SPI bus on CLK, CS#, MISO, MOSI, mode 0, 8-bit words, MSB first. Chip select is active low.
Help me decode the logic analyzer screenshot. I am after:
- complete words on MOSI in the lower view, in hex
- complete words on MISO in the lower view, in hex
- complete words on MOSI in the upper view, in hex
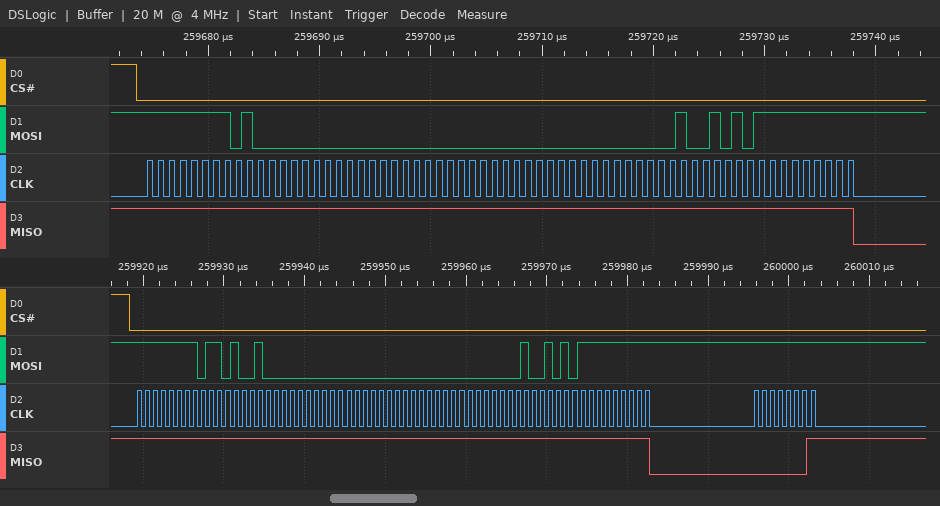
FF, 69, 00, 00, 00, 00, 95, FF, FF
FF, FF, FF, FF, FF, FF, FF, FF, 01
FF, 40, 00, 00, 00, 00, 95, FF
